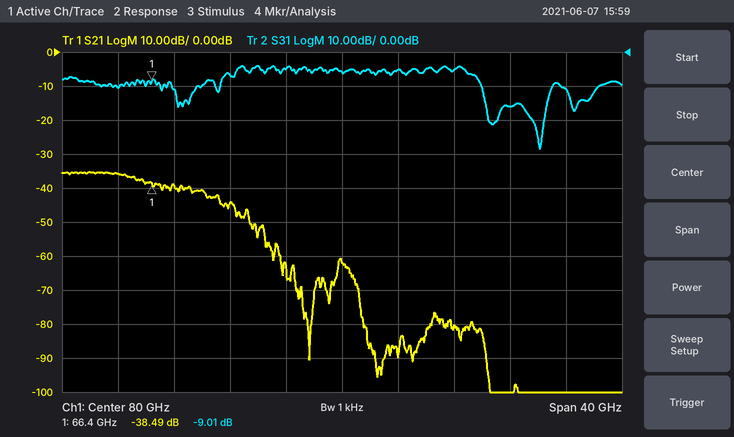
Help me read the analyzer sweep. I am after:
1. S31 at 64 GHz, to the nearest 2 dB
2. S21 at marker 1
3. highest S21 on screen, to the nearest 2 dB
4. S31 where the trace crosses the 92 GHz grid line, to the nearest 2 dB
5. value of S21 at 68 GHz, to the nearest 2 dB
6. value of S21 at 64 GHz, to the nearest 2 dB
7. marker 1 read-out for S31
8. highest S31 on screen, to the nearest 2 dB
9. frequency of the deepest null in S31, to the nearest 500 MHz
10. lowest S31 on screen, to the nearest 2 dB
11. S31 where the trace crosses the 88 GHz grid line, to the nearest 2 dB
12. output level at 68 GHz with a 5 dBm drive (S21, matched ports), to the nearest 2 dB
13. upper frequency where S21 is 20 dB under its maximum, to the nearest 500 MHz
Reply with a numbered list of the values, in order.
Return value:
1. -10 dB
2. -38.49 dB
3. -36 dB
4. -16 dB
5. -40 dB
6. -36 dB
7. -9.01 dB
8. -4 dB
9. 94.0 GHz
10. -28 dB
11. -6 dB
12. -34 dBm
13. 74.5 GHz
